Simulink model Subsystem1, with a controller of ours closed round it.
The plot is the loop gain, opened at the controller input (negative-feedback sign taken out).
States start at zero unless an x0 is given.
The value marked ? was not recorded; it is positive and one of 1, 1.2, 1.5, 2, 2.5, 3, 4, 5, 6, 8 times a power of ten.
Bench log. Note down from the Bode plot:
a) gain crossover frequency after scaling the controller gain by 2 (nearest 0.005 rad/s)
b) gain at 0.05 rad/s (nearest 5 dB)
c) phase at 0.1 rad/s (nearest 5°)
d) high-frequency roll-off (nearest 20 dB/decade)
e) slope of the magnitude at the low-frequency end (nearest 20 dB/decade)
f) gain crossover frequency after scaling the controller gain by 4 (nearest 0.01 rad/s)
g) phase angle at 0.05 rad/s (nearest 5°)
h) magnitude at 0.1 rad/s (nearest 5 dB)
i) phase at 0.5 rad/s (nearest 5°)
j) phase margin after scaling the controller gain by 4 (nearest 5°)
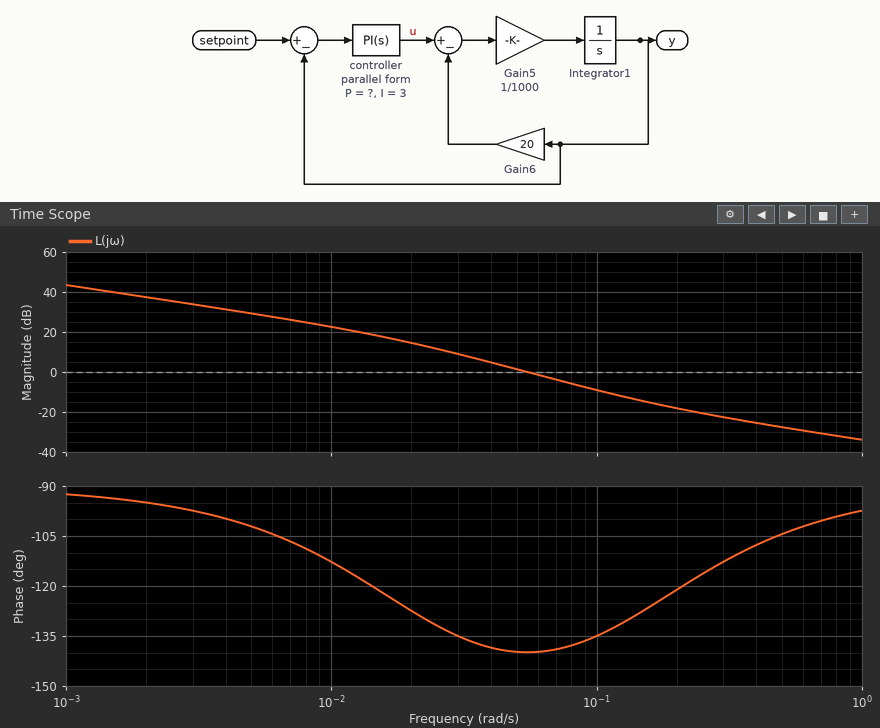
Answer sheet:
0.080 rad/s
0 dB
-135°
-20 dB/decade
-20 dB/decade
0.12 rad/s
-140°
-10 dB
-105°
50°
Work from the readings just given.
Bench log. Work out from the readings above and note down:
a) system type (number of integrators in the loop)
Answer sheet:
1
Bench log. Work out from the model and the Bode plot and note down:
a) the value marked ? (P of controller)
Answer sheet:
20
